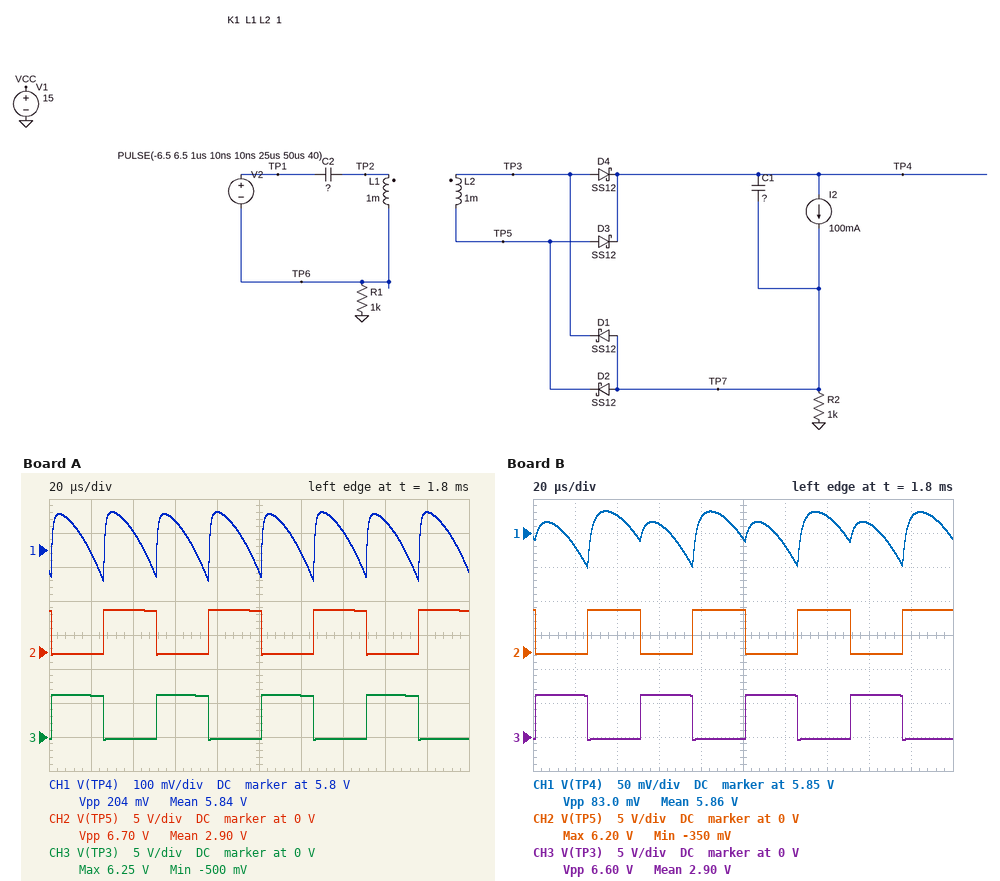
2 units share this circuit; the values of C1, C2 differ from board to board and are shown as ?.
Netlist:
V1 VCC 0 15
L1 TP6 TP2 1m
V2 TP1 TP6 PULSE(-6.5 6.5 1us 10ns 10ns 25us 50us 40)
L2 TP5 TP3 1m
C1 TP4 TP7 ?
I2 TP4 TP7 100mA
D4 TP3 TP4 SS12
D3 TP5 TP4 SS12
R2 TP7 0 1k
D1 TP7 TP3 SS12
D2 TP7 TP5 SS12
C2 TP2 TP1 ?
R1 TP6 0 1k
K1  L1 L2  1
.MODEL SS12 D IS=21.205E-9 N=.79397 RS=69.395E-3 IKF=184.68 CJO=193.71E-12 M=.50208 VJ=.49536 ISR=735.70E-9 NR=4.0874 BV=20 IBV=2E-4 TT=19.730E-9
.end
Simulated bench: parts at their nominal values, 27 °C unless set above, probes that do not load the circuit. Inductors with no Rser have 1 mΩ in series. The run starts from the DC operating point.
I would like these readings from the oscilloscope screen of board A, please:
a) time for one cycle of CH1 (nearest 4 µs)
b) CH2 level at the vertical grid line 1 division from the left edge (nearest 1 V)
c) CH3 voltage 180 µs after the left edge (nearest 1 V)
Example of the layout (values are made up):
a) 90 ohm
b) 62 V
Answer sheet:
a) 24 µs
b) 0 V
c) 0 V
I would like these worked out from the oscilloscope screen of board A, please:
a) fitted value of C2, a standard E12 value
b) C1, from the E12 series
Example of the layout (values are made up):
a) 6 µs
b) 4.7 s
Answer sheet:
a) 6.8 µF
b) 3.9 µF
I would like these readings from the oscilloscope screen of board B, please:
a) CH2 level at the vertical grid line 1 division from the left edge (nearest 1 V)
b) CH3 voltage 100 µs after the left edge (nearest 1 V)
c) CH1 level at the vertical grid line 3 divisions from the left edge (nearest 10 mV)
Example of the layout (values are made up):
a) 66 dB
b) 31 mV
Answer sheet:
a) 0 V
b) 0 V
c) 5.86 V
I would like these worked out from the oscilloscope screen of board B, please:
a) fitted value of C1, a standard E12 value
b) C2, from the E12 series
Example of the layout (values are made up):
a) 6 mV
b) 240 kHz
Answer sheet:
a) 12 µF
b) 15 µF
